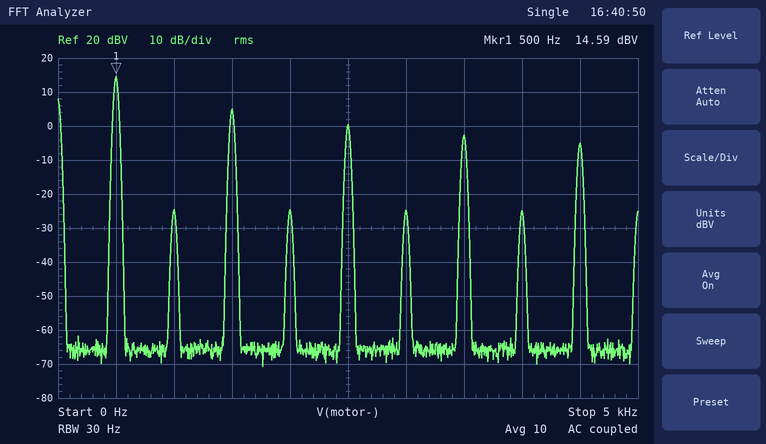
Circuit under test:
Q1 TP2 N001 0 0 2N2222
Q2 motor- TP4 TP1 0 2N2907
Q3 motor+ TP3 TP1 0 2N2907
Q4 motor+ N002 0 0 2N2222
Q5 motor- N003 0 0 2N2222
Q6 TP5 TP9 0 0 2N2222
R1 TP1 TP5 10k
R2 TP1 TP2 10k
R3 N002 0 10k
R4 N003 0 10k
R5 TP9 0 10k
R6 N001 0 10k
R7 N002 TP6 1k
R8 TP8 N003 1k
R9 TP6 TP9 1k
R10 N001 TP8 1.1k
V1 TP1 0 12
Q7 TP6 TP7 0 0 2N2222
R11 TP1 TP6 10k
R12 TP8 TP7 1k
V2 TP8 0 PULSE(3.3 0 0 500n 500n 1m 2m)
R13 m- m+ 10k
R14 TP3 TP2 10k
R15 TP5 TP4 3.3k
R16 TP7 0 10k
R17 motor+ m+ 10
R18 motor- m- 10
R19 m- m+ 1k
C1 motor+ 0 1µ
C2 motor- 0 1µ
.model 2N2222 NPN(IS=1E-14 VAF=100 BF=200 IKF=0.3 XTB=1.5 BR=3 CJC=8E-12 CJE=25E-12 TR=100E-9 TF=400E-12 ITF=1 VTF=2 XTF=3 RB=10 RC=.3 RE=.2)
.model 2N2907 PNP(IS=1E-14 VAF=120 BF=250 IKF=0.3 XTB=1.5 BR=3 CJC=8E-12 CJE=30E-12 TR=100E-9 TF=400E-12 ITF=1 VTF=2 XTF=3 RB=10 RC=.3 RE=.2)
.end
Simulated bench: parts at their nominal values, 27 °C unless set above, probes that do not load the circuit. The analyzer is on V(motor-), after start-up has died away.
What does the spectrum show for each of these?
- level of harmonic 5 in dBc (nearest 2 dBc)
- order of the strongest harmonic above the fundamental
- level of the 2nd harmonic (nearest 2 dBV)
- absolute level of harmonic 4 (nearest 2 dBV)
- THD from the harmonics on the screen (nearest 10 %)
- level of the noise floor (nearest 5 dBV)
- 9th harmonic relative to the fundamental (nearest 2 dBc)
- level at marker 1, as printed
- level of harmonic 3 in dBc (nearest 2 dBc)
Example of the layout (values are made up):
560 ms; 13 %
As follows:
-14 dBc; 3; -24 dBV; -24 dBV; 40 %; -65 dBV; -20 dBc; 14.59 dBV; -10 dBc
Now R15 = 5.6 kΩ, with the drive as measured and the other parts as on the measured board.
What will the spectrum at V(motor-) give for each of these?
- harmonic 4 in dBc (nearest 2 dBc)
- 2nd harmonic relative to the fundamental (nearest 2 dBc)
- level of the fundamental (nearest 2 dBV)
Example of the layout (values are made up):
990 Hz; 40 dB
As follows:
-56 dBc; -56 dBc; 14 dBV
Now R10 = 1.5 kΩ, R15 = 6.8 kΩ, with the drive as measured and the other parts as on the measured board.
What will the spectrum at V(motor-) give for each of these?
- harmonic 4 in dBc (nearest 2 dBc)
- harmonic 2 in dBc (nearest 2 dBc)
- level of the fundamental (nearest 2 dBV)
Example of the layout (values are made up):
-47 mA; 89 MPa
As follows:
-50 dBc; -50 dBc; 14 dBV
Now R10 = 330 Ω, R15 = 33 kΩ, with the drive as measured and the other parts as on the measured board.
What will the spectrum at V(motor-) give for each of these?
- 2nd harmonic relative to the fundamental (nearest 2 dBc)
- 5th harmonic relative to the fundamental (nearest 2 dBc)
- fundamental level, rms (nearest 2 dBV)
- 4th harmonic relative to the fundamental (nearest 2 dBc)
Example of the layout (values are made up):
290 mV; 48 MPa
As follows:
-22 dBc; -16 dBc; 14 dBV; -22 dBc
